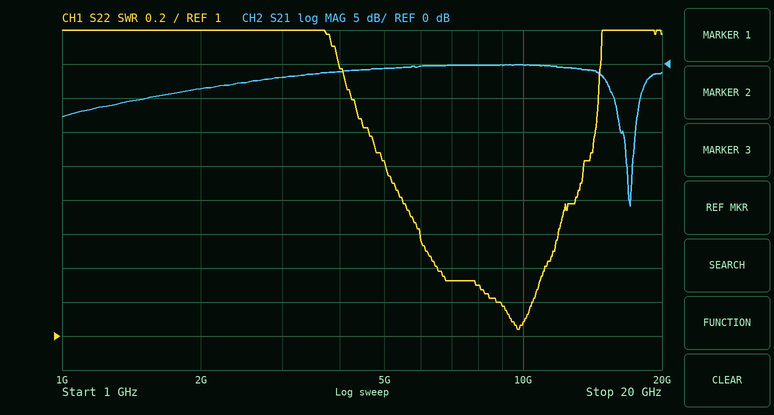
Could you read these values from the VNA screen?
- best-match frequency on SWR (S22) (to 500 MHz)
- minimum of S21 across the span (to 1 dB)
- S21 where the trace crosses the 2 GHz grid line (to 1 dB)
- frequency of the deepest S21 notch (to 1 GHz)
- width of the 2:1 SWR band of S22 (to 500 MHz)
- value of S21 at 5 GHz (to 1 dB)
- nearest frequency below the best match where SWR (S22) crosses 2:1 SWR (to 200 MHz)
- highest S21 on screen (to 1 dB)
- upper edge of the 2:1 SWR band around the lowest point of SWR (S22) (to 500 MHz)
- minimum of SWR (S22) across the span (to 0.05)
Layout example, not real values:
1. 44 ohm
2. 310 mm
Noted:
1. 9.5 GHz
2. -21 dB
3. -4 dB
4. 17 GHz
5. 8.5 GHz
6. -1 dB
7. 5.0 GHz
8. 0 dB
9. 13.5 GHz
10. 1.05
